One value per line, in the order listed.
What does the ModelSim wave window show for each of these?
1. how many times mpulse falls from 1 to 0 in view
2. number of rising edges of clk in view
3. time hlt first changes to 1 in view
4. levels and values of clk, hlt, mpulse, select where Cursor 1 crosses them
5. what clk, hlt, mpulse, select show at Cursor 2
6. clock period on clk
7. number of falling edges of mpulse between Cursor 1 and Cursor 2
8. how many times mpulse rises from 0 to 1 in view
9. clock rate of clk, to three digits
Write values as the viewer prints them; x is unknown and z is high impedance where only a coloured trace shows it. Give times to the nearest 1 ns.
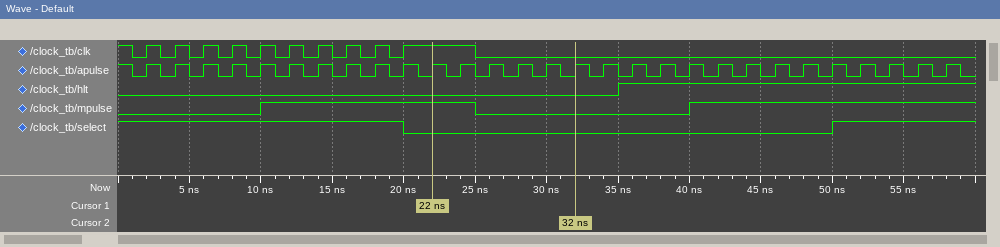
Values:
1
10
35 ns
clk=1, hlt=0, mpulse=1, select=0
clk=0, hlt=0, mpulse=0, select=0
2 ns
1
2
500 MHz
